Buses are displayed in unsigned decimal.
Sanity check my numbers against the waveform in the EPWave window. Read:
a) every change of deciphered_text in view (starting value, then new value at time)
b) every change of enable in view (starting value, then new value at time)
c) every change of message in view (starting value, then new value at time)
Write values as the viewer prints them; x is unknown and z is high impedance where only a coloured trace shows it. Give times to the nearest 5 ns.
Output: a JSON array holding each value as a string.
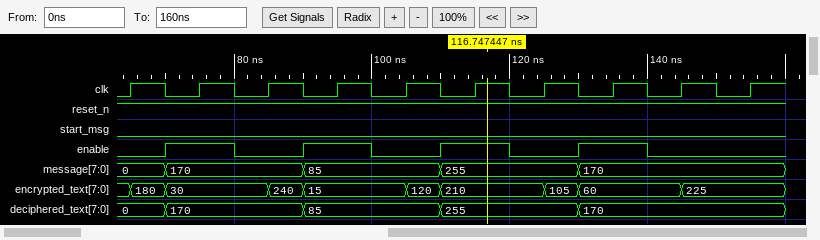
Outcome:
["0, 170 at 70 ns, 85 at 90 ns, 255 at 110 ns, 170 at 130 ns", "0, 1 at 70 ns, 0 at 80 ns, 1 at 90 ns, 0 at 100 ns, 1 at 110 ns, 0 at 120 ns, 1 at 130 ns, 0 at 140 ns", "0, 170 at 70 ns, 85 at 90 ns, 255 at 110 ns, 170 at 130 ns"]
